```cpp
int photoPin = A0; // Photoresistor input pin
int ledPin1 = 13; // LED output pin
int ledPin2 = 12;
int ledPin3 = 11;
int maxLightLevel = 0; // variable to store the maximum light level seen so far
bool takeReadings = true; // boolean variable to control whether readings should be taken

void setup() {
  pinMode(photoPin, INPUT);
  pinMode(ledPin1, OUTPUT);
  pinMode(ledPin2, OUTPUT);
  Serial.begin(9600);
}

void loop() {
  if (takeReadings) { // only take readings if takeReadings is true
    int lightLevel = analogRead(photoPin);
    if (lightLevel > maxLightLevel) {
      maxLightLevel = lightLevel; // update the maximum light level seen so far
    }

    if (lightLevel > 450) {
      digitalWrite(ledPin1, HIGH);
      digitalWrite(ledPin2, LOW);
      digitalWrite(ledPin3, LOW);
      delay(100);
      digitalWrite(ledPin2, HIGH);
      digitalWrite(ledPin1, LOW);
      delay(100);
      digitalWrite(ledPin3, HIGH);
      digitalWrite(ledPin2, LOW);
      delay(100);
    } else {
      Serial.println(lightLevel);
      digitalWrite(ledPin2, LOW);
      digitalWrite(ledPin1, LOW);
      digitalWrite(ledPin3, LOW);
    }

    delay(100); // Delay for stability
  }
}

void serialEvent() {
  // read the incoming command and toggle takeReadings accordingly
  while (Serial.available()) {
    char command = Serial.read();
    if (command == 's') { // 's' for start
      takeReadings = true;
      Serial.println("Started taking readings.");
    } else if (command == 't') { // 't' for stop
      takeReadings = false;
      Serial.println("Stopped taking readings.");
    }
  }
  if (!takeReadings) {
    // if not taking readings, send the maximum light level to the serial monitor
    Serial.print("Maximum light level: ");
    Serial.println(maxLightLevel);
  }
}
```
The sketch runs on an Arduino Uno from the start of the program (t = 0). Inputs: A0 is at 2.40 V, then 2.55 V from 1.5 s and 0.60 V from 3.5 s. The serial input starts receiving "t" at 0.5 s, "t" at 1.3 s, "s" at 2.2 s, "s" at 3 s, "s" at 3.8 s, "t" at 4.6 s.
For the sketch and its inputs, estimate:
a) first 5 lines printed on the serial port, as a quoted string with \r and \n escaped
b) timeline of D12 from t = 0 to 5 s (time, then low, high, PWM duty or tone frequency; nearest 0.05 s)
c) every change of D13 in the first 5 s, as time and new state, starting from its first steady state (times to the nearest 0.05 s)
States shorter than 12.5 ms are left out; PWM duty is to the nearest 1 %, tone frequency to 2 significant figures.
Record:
"Stopped taking readings.\r\nMaximum light level: 491\r\nStopped taking readings.\r\nMaximum light level: 491\r\nStarted taking readings.\r\n"
0 s low; 0.1 s high; 0.2 s low; 0.5 s high; 0.6 s low; 2.3 s high; 2.4 s low; 2.7 s high; 2.8 s low; 3.1 s high; 3.2 s low; 3.5 s high; 3.6 s low
0 s high; 0.1 s low; 0.4 s high; 0.5 s low; 2.2 s high; 2.3 s low; 2.6 s high; 2.7 s low; 3 s high; 3.1 s low; 3.4 s high; 3.5 s low
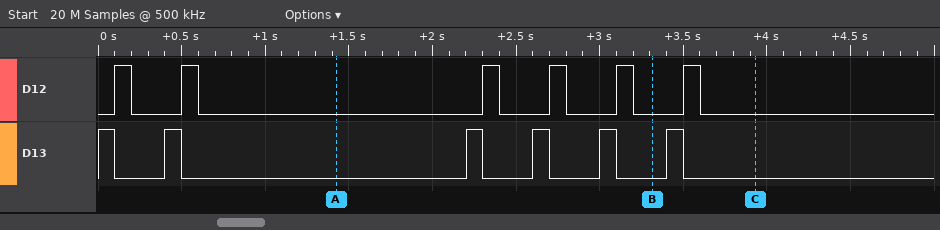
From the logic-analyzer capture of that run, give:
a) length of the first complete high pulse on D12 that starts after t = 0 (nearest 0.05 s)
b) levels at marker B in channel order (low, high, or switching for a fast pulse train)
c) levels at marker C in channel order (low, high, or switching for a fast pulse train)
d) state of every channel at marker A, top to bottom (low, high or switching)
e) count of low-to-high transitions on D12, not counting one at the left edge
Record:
0.10 s
D12 low, D13 low
D12 low, D13 low
D12 low, D13 low
6
